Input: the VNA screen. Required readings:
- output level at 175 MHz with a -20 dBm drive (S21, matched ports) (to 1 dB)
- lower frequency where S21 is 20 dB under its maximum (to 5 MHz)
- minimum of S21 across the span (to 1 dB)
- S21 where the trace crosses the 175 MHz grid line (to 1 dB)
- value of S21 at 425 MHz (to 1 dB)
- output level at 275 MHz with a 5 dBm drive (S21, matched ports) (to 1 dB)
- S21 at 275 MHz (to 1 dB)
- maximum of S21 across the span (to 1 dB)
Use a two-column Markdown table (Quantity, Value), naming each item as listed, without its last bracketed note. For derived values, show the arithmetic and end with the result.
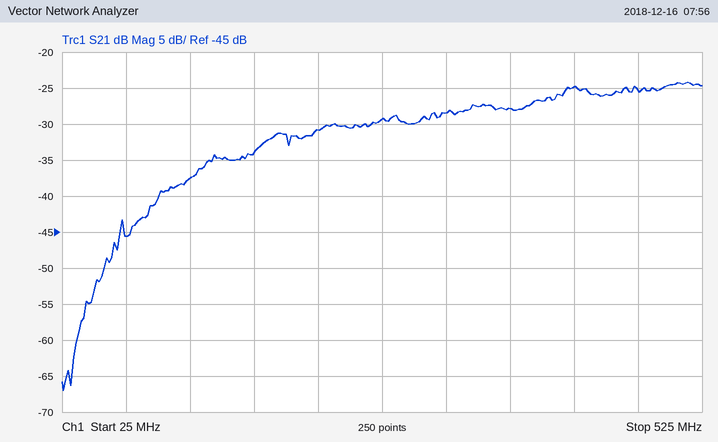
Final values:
| Quantity | Value |
|---|---|
| output level at 175 MHz with a -20 dBm drive (S21, matched ports) | -20 dBm + (-34 dB) = -54 dBm |
| lower frequency where S21 is 20 dB under its maximum | 80 MHz |
| minimum of S21 across the span | -67 dB |
| S21 where the trace crosses the 175 MHz grid line | -34 dB |
| value of S21 at 425 MHz | -25 dB |
| output level at 275 MHz with a 5 dBm drive (S21, matched ports) | 5 dBm + (-29 dB) = -24 dBm |
| S21 at 275 MHz | -29 dB |
| maximum of S21 across the span | -24 dB |
